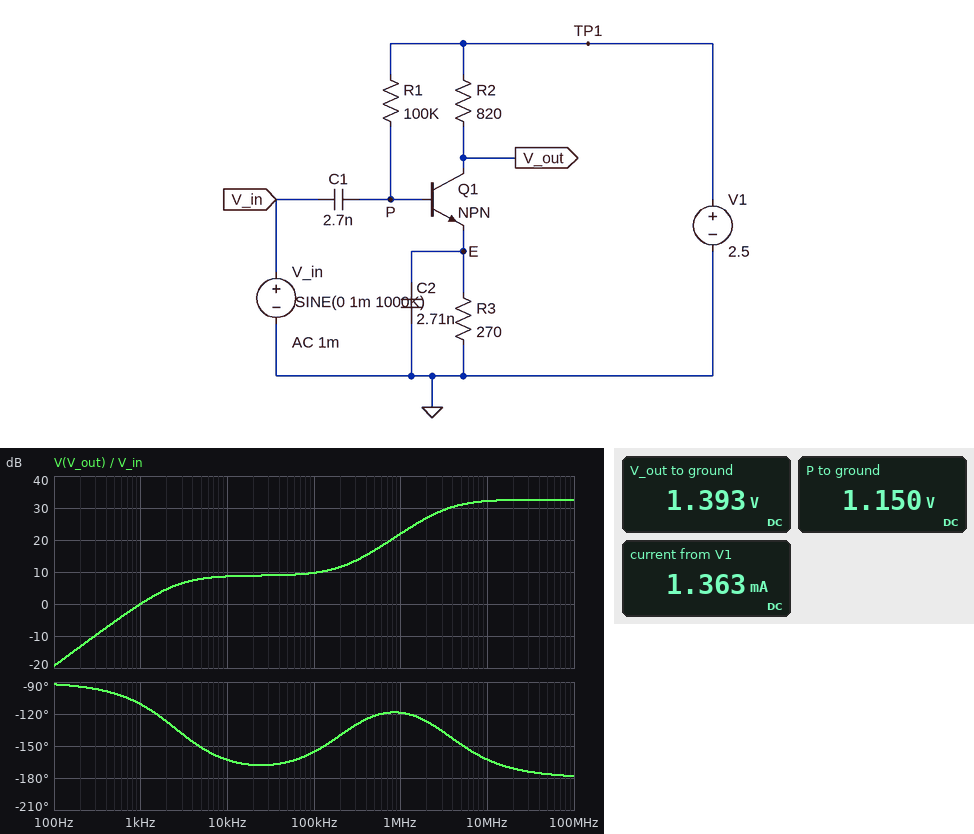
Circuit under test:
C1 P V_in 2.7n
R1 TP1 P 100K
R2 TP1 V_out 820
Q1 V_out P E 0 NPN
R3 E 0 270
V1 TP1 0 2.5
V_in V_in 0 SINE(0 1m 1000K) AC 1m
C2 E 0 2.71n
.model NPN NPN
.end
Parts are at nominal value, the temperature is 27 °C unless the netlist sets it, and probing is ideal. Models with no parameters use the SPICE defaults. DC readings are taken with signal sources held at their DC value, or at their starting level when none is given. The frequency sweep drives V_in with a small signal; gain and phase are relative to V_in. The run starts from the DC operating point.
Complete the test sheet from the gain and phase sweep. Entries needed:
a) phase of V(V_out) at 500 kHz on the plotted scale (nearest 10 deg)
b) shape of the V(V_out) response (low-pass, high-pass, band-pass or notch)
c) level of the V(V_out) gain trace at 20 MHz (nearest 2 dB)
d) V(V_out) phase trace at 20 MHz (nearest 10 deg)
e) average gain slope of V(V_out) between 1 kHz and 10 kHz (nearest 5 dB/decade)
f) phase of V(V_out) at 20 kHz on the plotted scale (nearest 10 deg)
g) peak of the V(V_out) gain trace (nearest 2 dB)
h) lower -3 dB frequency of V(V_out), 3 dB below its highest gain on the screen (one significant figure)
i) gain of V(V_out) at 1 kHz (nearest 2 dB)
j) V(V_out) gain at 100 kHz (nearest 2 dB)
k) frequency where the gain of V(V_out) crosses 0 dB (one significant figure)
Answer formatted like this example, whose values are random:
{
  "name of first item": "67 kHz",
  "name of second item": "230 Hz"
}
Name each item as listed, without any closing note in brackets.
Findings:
{
  "phase of V(V_out) at 500 kHz on the plotted scale": "-120 deg",
  "shape of the V(V_out) response": "high-pass",
  "level of the V(V_out) gain trace at 20 MHz": "32 dB",
  "V(V_out) phase trace at 20 MHz": "-170 deg",
  "average gain slope of V(V_out) between 1 kHz and 10 kHz": "10 dB/decade",
  "phase of V(V_out) at 20 kHz on the plotted scale": "-170 deg",
  "peak of the V(V_out) gain trace": "32 dB",
  "lower -3 dB frequency of V(V_out), 3 dB below its highest gain on the screen": "3 MHz",
  "gain of V(V_out) at 1 kHz": "0 dB",
  "V(V_out) gain at 100 kHz": "10 dB",
  "frequency where the gain of V(V_out) crosses 0 dB": "1 kHz"
}
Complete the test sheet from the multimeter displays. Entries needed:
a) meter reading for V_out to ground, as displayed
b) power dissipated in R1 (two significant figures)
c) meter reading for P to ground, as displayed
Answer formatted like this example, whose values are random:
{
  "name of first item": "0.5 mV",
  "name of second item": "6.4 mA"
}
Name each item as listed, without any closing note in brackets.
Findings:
{
  "meter reading for V_out to ground, as displayed": "1.393 V",
  "power dissipated in R1": "18 µW",
  "meter reading for P to ground, as displayed": "1.150 V"
}
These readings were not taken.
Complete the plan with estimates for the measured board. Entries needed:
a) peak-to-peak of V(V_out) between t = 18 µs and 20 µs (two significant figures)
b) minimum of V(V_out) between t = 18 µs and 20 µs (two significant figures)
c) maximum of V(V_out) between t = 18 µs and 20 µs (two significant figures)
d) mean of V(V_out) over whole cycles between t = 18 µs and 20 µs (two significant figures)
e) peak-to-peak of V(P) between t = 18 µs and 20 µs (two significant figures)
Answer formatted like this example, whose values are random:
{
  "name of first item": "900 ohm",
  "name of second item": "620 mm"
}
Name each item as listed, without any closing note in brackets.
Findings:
{
  "peak-to-peak of V(V_out) between t = 18 µs and 20 µs": "25 mV",
  "minimum of V(V_out) between t = 18 µs and 20 µs": "1.4 V",
  "maximum of V(V_out) between t = 18 µs and 20 µs": "1.4 V",
  "mean of V(V_out) over whole cycles between t = 18 µs and 20 µs": "1.4 V",
  "peak-to-peak of V(P) between t = 18 µs and 20 µs": "2.0 mV"
}
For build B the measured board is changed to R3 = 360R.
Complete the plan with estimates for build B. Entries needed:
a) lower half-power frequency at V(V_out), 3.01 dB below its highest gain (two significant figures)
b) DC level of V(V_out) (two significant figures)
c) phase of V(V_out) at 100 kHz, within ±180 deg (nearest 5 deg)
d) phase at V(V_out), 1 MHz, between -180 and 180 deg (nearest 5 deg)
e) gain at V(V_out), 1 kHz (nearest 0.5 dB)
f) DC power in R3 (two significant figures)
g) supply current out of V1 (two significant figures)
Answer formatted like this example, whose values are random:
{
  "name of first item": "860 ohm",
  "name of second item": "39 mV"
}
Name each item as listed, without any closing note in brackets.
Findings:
{
  "lower half-power frequency at V(V_out), 3.01 dB below its highest gain": "3.1 MHz",
  "DC level of V(V_out)": "1.5 V",
  "phase of V(V_out) at 100 kHz, within ±180 deg": "-150 deg",
  "phase at V(V_out), 1 MHz, between -180 and 180 deg": "-115 deg",
  "gain at V(V_out), 1 kHz": "-1.0 dB",
  "DC power in R3": "580 µW",
  "supply current out of V1": "1.3 mA"
}
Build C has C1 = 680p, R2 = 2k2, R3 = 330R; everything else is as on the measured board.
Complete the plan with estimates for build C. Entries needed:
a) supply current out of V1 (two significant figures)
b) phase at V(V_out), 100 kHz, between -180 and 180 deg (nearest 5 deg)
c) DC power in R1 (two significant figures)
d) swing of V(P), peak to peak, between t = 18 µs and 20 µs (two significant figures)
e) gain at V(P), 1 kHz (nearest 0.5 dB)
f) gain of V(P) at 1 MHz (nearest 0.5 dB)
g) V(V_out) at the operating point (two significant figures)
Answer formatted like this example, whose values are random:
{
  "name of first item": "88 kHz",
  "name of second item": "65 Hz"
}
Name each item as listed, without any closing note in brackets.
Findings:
{
  "supply current out of V1": "950 µA",
  "phase at V(V_out), 100 kHz, between -180 and 180 deg": "-105 deg",
  "DC power in R1": "20 µW",
  "swing of V(P), peak to peak, between t = 18 µs and 20 µs": "1.1 mV",
  "gain at V(P), 1 kHz": "-47.0 dB",
  "gain of V(P) at 1 MHz": "-5.5 dB",
  "V(V_out) at the operating point": "450 mV"
}
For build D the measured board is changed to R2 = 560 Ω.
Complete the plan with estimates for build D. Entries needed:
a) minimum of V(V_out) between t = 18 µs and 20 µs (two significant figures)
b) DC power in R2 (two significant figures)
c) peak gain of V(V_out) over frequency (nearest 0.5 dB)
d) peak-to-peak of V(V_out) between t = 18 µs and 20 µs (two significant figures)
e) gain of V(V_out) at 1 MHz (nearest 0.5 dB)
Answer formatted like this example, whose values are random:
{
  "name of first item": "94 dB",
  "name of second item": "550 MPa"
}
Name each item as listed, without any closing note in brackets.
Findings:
{
  "minimum of V(V_out) between t = 18 µs and 20 µs": "1.7 V",
  "DC power in R2": "1.0 mW",
  "peak gain of V(V_out) over frequency": "29.5 dB",
  "peak-to-peak of V(V_out) between t = 18 µs and 20 µs": "17 mV",
  "gain of V(V_out) at 1 MHz": "18.5 dB"
}
